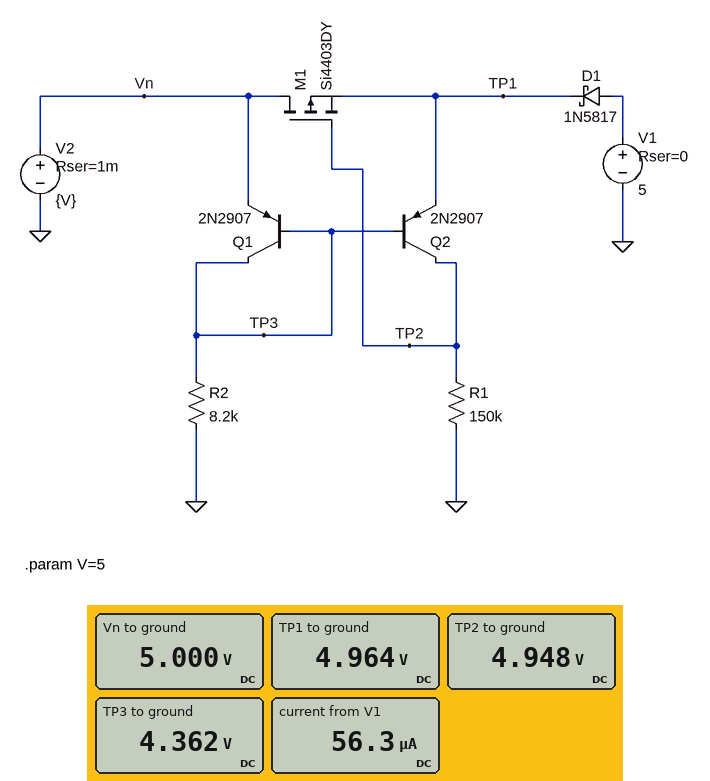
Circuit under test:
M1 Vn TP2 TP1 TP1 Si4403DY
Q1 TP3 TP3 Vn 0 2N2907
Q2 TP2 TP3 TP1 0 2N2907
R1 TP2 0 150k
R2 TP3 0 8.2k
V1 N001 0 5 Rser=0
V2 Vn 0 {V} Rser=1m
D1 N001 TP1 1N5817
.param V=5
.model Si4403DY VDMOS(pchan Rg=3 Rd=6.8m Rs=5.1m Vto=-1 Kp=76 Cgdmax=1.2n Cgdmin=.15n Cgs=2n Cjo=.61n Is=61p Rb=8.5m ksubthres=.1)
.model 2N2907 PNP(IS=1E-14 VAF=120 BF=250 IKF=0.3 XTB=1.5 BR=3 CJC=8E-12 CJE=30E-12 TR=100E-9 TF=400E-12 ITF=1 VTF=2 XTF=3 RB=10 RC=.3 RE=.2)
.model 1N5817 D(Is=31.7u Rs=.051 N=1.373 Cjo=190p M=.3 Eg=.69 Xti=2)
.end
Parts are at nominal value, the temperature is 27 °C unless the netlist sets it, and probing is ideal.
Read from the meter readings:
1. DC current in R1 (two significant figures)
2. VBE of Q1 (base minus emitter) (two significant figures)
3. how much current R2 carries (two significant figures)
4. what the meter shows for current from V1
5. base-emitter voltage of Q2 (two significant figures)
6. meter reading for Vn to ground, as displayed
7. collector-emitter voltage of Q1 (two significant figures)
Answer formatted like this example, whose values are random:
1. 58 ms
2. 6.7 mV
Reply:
1. 33 µA
2. -640 mV
3. 530 µA
4. 56.3 µA
5. -600 mV
6. 5.000 V
7. -640 mV
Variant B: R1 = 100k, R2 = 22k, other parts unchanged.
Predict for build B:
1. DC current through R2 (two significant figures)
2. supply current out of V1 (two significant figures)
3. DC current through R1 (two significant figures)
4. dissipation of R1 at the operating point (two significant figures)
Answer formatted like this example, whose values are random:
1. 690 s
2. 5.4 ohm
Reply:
1. 200 µA
2. 50 µA
3. 49 µA
4. 240 µW
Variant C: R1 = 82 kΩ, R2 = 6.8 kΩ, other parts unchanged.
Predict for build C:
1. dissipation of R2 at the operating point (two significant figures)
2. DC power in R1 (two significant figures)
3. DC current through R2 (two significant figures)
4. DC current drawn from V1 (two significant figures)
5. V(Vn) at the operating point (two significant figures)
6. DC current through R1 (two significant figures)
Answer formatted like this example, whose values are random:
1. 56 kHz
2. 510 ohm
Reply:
1. 2.8 mW
2. 300 µW
3. 640 µA
4. 75 µA
5. 5.0 V
6. 60 µA
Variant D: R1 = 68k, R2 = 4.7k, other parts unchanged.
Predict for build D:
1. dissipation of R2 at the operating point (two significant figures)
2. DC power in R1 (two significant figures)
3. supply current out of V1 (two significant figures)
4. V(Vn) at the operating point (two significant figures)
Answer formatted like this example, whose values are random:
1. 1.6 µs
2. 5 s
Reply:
1. 4.0 mW
2. 360 µW
3. 90 µA
4. 5.0 V
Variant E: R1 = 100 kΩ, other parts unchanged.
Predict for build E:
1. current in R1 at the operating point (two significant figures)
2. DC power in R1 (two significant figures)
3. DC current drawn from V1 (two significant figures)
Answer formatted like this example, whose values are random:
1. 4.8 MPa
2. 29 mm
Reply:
1. 49 µA
2. 240 µW
3. 65 µA
